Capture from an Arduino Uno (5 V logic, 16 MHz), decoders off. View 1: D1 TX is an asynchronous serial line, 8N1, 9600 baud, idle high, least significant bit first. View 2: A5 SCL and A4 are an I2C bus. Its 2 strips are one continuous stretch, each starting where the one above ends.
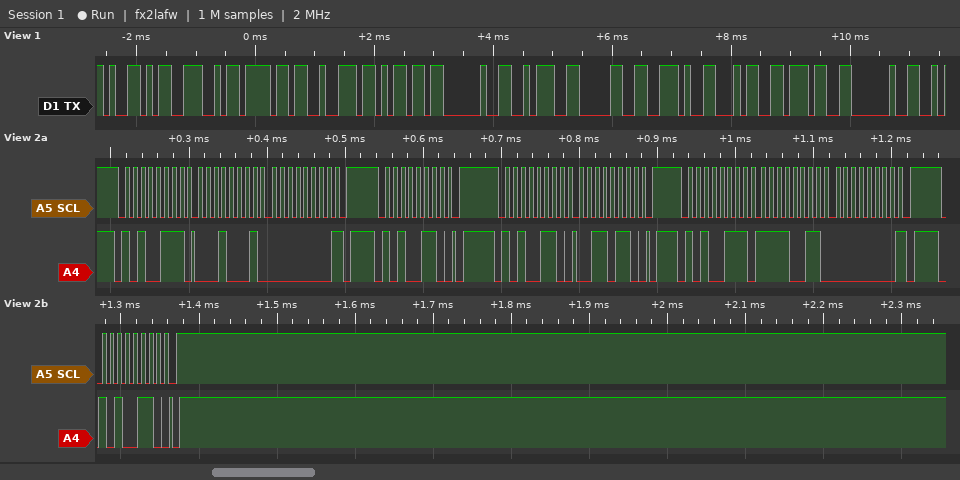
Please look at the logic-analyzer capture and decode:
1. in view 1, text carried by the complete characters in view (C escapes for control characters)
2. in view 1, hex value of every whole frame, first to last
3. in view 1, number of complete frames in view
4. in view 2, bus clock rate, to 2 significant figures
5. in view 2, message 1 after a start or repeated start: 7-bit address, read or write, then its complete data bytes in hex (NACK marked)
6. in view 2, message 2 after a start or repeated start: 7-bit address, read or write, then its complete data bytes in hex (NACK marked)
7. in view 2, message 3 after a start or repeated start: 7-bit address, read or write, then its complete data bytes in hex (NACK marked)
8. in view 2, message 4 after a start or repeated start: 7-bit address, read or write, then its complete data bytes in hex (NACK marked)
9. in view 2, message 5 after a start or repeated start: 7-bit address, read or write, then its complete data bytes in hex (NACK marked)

"YNorm :0.47 "
59 4E 6F 72 6D 20 3A 30 2E 34 37 20
12
100 kHz
0x53 read: 11 00 NACK
0x53 write
0x53 write: 36
0x53 read: F3 00 NACK
0x53 write
